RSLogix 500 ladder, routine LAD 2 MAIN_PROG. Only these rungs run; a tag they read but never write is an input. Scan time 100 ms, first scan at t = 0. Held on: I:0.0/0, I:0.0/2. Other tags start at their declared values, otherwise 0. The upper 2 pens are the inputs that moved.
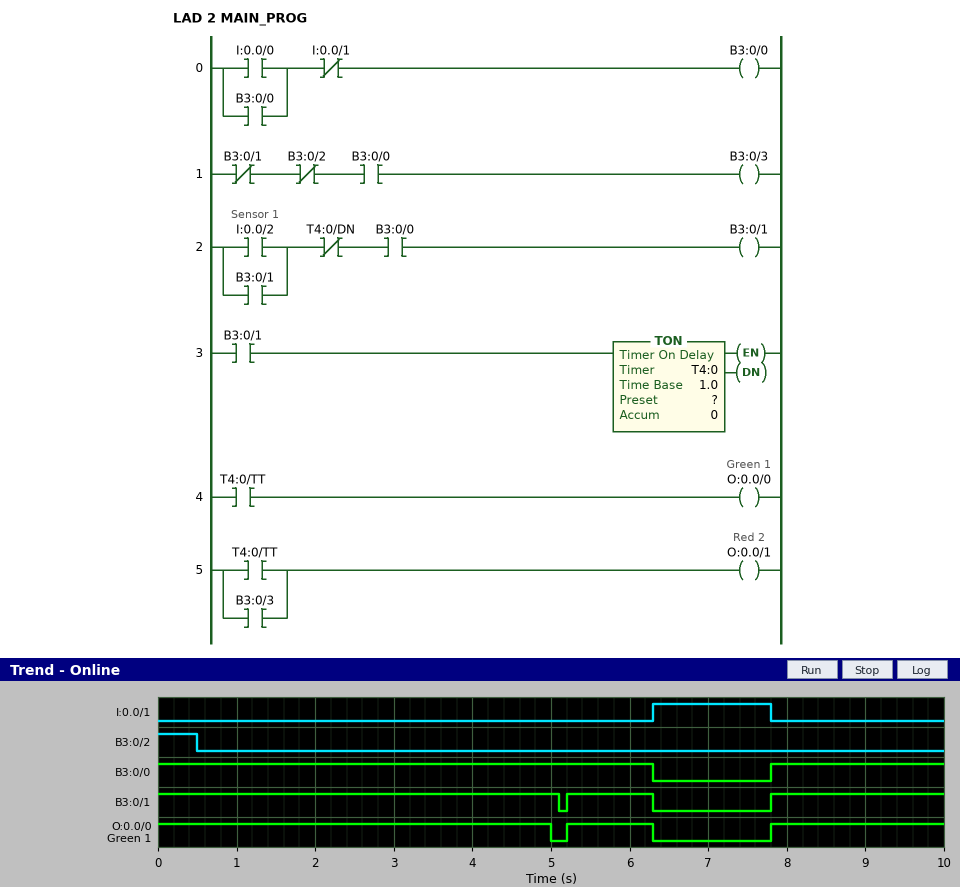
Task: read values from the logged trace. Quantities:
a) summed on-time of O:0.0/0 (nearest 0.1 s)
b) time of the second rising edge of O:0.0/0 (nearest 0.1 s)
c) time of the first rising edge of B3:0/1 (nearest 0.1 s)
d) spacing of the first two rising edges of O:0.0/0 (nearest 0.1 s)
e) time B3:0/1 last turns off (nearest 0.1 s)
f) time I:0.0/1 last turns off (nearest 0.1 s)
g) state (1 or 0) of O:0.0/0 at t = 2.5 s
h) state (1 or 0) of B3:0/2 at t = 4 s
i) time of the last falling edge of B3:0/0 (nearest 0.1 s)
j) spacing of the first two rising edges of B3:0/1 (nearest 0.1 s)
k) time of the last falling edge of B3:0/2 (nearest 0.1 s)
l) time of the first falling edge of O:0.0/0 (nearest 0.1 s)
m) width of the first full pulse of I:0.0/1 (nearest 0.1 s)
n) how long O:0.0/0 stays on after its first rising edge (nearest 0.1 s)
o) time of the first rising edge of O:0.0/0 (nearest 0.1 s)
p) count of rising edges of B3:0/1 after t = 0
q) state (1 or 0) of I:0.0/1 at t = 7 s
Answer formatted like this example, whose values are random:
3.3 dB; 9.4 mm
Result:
8.3 s; 7.8 s; 5.2 s; 2.6 s; 6.3 s; 7.8 s; 1; 0; 6.3 s; 2.6 s; 0.5 s; 5.0 s; 1.5 s; 1.1 s; 5.2 s; 2; 1
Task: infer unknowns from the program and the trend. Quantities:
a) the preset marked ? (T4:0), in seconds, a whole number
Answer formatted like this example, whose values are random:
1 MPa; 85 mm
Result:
5 s
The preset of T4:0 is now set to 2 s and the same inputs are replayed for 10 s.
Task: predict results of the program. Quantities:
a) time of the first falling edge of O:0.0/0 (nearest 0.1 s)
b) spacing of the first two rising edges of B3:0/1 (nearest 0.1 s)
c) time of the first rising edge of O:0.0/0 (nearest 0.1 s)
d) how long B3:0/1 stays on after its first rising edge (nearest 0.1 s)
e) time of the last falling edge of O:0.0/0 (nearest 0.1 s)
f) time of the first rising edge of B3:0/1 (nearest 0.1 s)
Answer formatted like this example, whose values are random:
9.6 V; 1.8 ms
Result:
2.0 s; 2.2 s; 2.2 s; 2.1 s; 9.8 s; 2.2 s
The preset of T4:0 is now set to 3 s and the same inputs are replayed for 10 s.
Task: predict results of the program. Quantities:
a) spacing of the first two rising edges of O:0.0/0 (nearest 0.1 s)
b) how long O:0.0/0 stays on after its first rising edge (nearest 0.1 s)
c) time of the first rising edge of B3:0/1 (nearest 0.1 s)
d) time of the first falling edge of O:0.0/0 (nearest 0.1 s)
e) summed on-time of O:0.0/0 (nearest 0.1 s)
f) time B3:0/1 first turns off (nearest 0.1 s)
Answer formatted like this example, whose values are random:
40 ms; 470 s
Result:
4.6 s; 3.0 s; 3.2 s; 3.0 s; 8.2 s; 3.1 s
